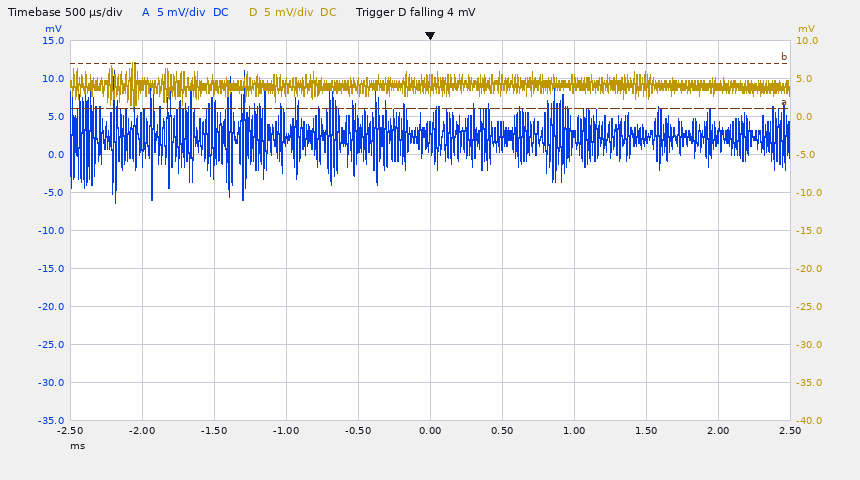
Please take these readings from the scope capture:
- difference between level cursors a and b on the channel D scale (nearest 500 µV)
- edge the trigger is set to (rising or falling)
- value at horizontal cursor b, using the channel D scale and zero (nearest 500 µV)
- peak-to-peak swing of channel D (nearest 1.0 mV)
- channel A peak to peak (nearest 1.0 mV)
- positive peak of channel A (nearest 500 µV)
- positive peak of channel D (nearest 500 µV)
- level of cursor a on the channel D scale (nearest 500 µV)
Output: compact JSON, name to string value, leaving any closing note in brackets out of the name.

{"difference between level cursors a and b on the channel D scale": "6.0 mV", "edge the trigger is set to": "falling", "value at horizontal cursor b, using the channel D scale and zero": "7.0 mV", "peak-to-peak swing of channel D": "6.0 mV", "channel A peak to peak": "17.0 mV", "positive peak of channel A": "11.0 mV", "positive peak of channel D": "7.0 mV", "level of cursor a on the channel D scale": "1.0 mV"}
